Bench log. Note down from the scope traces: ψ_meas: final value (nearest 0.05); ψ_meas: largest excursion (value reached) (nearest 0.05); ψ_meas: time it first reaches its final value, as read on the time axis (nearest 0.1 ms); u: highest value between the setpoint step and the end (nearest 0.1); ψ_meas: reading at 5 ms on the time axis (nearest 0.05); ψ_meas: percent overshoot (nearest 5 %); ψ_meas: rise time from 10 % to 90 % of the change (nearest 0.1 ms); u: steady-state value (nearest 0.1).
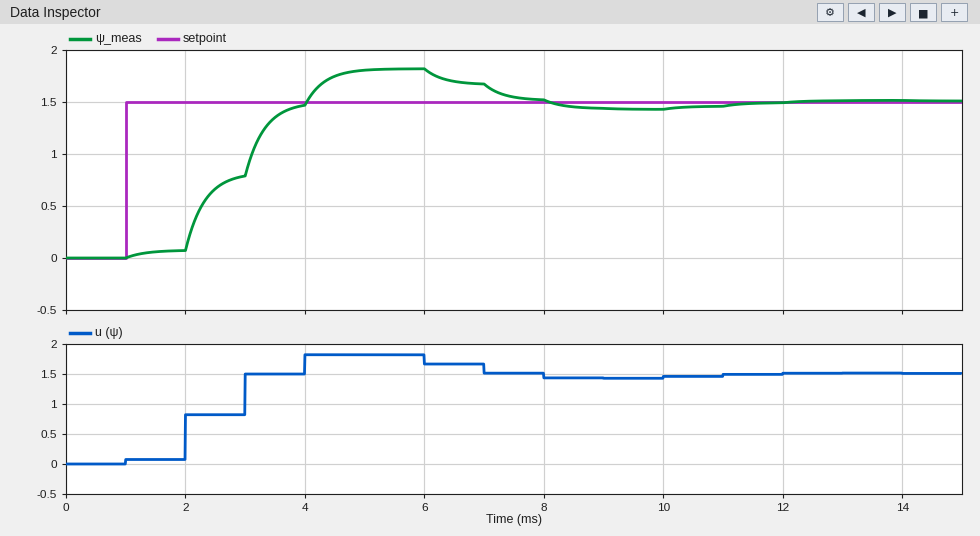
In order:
1.50
1.80
4.0 ms
1.8
1.80
20 %
1.5 ms
1.5
